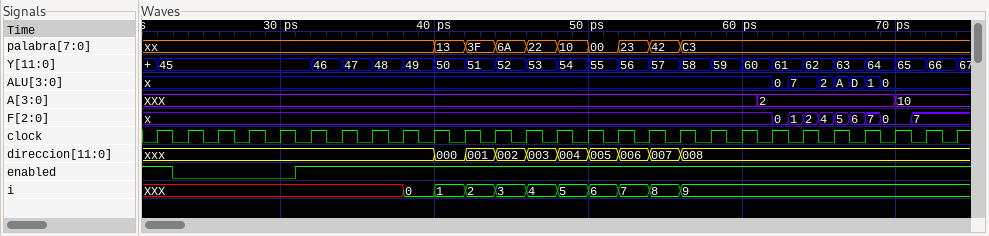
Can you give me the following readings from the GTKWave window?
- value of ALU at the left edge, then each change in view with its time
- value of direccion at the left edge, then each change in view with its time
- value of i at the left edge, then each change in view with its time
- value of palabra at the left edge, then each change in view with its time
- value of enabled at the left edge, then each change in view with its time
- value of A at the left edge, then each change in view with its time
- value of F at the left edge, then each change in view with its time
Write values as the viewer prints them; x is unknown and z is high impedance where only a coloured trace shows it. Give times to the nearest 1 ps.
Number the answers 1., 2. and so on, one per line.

1. x, 0 at 62 ps, 7 at 63 ps, 2 at 65 ps, A at 66 ps, D at 67 ps, 1 at 68 ps, 0 at 69 ps
2. xxx, 000 at 40 ps, 001 at 42 ps, 002 at 44 ps, 003 at 46 ps, 004 at 48 ps, 005 at 50 ps, 006 at 52 ps, 007 at 54 ps, 008 at 56 ps
3. XXX, 0 at 38 ps, 1 at 40 ps, 2 at 42 ps, 3 at 44 ps, 4 at 46 ps, 5 at 48 ps, 6 at 50 ps, 7 at 52 ps, 8 at 54 ps, 9 at 56 ps
4. xx, 13 at 40 ps, 3F at 42 ps, 6A at 44 ps, 22 at 46 ps, 10 at 48 ps, 00 at 50 ps, 23 at 52 ps, 42 at 54 ps, C3 at 56 ps
5. 1, 0 at 23 ps, 1 at 31 ps
6. XXX, 2 at 61 ps, 10 at 70 ps
7. x, 0 at 62 ps, 1 at 63 ps, 2 at 64 ps, 4 at 65 ps, 5 at 66 ps, 6 at 67 ps, 7 at 68 ps, 0 at 69 ps, 7 at 71 ps
